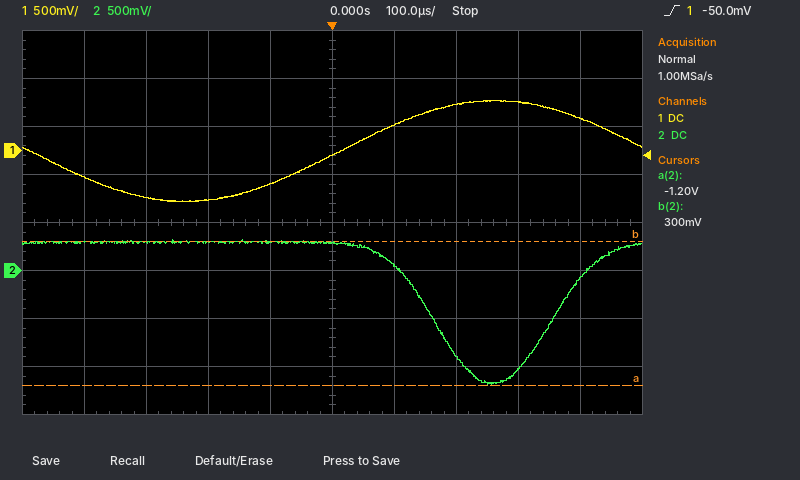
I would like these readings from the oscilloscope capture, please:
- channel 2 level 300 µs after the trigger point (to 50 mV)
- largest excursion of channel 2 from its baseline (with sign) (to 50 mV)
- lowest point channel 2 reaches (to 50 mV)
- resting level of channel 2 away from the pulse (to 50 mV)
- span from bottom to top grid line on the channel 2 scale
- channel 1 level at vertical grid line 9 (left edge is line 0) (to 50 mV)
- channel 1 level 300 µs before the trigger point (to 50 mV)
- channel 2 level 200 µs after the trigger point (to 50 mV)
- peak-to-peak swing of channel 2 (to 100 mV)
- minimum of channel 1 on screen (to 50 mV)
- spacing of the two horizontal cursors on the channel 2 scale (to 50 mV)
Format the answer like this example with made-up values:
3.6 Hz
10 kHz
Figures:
-1.05 V
-1.50 V
-1.20 V
300 mV
4 V
350 mV
-500 mV
-900 mV
1.50 V
-550 mV
1.50 V
